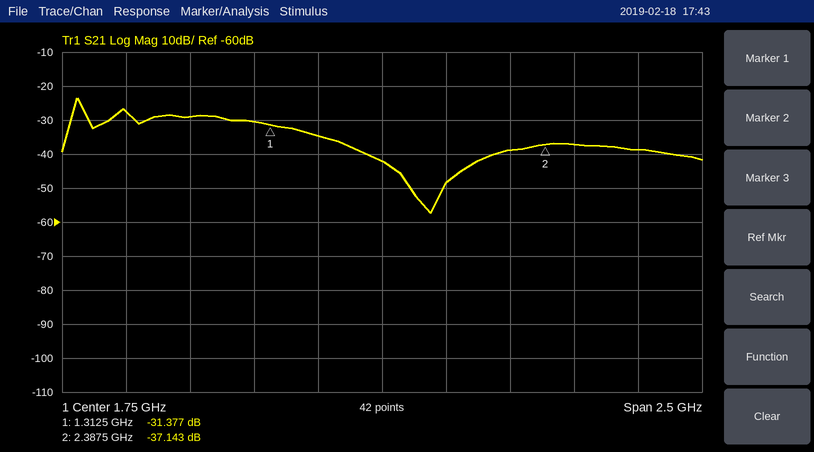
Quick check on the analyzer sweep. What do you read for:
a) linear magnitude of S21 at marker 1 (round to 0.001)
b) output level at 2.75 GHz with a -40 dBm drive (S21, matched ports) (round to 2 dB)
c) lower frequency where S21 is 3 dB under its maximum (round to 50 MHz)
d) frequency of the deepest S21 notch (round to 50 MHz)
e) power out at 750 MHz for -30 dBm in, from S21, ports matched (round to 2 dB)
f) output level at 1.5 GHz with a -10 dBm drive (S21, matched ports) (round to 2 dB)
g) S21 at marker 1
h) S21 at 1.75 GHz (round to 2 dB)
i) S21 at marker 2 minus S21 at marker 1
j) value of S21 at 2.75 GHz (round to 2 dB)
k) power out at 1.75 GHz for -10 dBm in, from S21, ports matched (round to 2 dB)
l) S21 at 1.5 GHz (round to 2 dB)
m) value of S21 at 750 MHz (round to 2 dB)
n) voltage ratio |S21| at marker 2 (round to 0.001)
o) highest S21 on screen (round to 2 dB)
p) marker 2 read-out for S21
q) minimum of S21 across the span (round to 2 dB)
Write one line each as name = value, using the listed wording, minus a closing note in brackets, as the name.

linear magnitude of S21 at marker 1 = 0.027
output level at 2.75 GHz with a -40 dBm drive (S21, matched ports) = -78 dBm
lower frequency where S21 is 3 dB under its maximum = 550 MHz
frequency of the deepest S21 notch = 1.95 GHz
power out at 750 MHz for -30 dBm in, from S21, ports matched = -58 dBm
output level at 1.5 GHz with a -10 dBm drive (S21, matched ports) = -44 dBm
S21 at marker 1 = -31.377 dB
S21 at 1.75 GHz = -42 dB
S21 at marker 2 minus S21 at marker 1 = -5.766 dB
value of S21 at 2.75 GHz = -38 dB
power out at 1.75 GHz for -10 dBm in, from S21, ports matched = -52 dBm
S21 at 1.5 GHz = -34 dB
value of S21 at 750 MHz = -28 dB
voltage ratio |S21| at marker 2 = 0.014
highest S21 on screen = -24 dB
marker 2 read-out for S21 = -37.143 dB
minimum of S21 across the span = -58 dB
